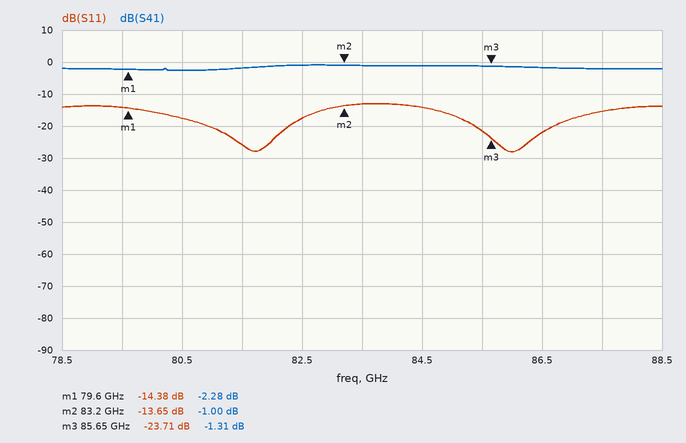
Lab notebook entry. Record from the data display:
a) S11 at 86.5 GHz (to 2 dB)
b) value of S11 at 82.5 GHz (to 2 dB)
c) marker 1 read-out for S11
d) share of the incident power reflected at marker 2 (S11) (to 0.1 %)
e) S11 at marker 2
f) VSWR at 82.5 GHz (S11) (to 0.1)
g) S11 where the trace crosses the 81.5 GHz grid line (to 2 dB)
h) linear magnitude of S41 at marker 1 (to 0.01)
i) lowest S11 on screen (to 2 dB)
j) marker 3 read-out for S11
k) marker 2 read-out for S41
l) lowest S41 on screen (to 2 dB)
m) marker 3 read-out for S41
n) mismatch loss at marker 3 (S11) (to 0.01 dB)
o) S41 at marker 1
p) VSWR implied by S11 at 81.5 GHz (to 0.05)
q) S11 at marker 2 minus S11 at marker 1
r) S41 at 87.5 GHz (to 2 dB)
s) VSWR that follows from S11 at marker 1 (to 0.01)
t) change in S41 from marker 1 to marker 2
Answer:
-22 dB
-18 dB
-14.38 dB
4.3 %
-13.65 dB
1.3
-26 dB
0.77
-28 dB
-23.71 dB
-1.00 dB
-2 dB
-1.31 dB
0.02 dB
-2.28 dB
1.10
0.73 dB
-2 dB
1.47
1.28 dB
